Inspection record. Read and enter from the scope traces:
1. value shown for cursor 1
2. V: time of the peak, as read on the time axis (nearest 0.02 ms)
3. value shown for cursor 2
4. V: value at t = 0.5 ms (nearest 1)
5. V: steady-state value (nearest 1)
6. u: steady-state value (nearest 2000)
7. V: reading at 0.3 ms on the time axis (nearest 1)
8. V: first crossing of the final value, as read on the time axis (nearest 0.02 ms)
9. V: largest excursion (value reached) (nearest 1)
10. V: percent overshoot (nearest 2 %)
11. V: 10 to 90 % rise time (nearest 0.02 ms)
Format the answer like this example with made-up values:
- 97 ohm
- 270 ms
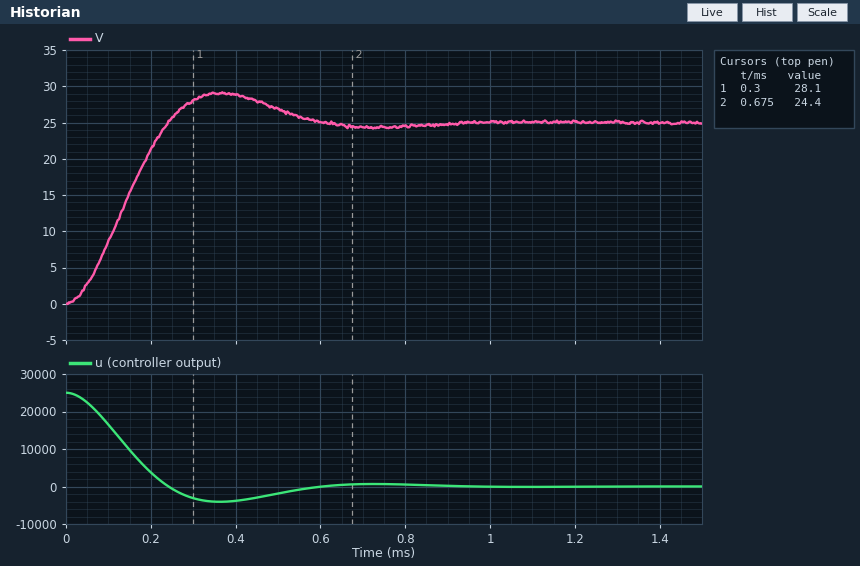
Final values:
- 28.1
- 0.36 ms
- 24.4
- 27
- 25
- 0
- 28
- 0.24 ms
- 29
- 16 %
- 0.16 ms
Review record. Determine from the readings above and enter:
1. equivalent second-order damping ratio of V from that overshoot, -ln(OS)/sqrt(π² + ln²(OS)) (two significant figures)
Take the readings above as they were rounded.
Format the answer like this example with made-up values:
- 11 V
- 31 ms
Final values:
- 0.50
